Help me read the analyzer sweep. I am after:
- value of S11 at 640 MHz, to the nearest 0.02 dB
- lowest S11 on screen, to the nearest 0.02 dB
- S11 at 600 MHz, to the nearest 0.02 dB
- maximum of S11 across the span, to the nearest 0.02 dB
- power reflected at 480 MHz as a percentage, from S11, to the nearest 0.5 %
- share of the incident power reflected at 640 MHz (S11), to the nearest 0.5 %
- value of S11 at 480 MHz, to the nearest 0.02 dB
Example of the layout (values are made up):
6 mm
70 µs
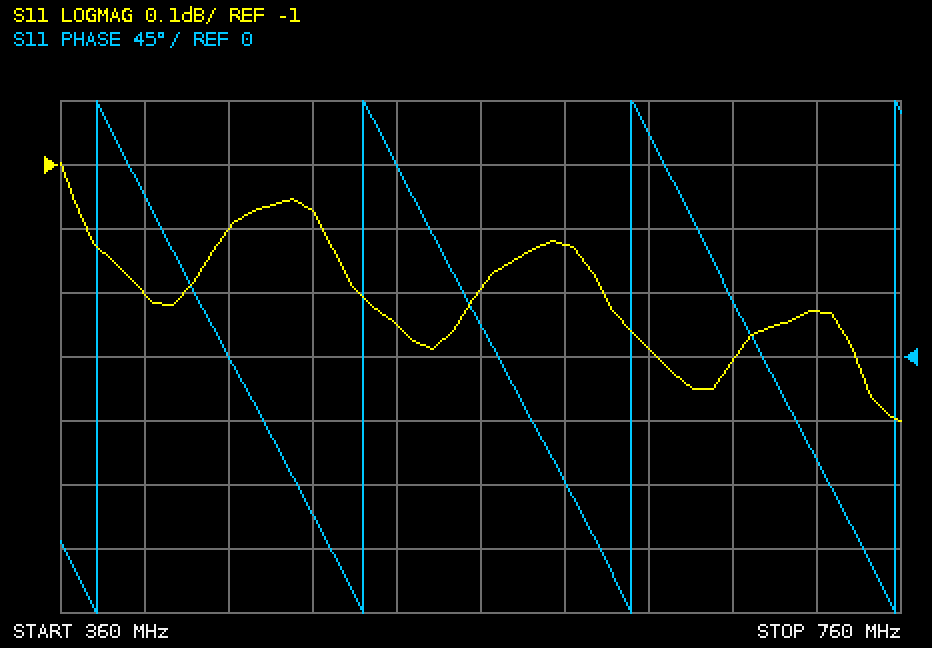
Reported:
-1.28 dB
-1.40 dB
-1.12 dB
-1.00 dB
78.0 %
74.5 %
-1.08 dB
